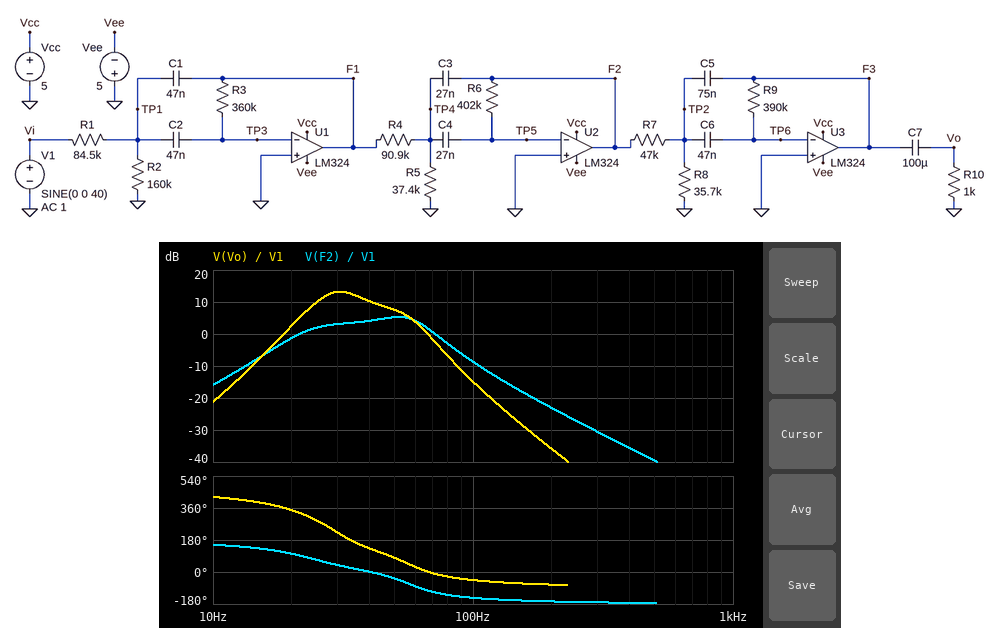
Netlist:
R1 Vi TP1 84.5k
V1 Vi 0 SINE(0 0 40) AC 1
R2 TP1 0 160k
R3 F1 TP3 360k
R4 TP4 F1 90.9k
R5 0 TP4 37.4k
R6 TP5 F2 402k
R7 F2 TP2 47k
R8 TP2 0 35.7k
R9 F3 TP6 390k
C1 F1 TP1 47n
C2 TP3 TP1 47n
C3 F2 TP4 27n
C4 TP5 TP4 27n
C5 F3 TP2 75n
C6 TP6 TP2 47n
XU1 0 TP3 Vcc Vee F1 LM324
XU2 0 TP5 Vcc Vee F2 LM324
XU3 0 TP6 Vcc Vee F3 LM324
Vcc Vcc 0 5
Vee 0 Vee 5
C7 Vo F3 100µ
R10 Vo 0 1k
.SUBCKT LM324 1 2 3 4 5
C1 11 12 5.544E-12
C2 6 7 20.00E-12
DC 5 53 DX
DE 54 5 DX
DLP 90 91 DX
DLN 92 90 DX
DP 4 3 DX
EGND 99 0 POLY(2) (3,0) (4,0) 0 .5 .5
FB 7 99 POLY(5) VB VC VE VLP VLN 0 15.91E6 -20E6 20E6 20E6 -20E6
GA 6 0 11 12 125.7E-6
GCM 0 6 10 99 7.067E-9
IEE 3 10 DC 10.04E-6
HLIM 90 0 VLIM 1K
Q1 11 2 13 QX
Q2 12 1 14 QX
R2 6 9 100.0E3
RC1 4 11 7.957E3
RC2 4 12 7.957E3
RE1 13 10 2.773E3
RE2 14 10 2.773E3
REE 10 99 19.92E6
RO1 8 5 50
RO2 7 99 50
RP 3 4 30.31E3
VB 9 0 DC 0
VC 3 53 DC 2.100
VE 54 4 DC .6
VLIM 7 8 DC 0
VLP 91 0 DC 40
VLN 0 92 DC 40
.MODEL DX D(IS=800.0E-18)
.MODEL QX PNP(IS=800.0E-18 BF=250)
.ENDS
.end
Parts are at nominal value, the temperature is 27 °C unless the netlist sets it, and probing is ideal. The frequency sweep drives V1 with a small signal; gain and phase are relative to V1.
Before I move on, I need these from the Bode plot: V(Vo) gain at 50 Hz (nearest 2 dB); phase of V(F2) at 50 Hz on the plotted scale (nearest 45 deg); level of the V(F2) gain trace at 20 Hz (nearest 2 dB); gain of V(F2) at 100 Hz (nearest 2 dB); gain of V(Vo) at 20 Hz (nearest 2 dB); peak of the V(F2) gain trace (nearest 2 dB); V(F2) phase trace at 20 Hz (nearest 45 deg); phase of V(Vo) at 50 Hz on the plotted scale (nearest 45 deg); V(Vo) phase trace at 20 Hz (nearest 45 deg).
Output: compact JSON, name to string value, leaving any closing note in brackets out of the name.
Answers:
{"V(Vo) gain at 50 Hz": "8 dB", "phase of V(F2) at 50 Hz on the plotted scale": "-45 deg", "level of the V(F2) gain trace at 20 Hz": "-2 dB", "gain of V(F2) at 100 Hz": "-8 dB", "gain of V(Vo) at 20 Hz": "2 dB", "peak of the V(F2) gain trace": "6 dB", "V(F2) phase trace at 20 Hz": "90 deg", "phase of V(Vo) at 50 Hz on the plotted scale": "90 deg", "V(Vo) phase trace at 20 Hz": "360 deg"}
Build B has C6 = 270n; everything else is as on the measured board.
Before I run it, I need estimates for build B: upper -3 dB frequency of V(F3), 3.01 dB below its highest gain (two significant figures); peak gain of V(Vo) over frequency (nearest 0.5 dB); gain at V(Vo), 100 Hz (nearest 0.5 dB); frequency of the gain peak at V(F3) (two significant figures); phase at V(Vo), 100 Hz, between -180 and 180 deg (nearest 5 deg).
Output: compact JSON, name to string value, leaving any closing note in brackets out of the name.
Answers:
{"upper -3 dB frequency of V(F3), 3.01 dB below its highest gain": "38 Hz", "peak gain of V(Vo) over frequency": "9.0 dB", "gain at V(Vo), 100 Hz": "-15.5 dB", "frequency of the gain peak at V(F3)": "23 Hz", "phase at V(Vo), 100 Hz, between -180 and 180 deg": "-50 deg"}
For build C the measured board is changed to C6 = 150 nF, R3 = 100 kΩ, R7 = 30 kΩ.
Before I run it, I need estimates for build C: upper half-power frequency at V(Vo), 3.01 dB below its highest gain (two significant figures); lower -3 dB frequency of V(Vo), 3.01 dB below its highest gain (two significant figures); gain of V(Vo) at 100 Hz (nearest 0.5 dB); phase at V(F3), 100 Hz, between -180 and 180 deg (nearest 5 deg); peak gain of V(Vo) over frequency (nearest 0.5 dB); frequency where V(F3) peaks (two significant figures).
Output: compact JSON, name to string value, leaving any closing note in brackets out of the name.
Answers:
{"upper half-power frequency at V(Vo), 3.01 dB below its highest gain": "64 Hz", "lower -3 dB frequency of V(Vo), 3.01 dB below its highest gain": "19 Hz", "gain of V(Vo) at 100 Hz": "-12.0 dB", "phase at V(F3), 100 Hz, between -180 and 180 deg": "-20 deg", "peak gain of V(Vo) over frequency": "5.5 dB", "frequency where V(F3) peaks": "51 Hz"}
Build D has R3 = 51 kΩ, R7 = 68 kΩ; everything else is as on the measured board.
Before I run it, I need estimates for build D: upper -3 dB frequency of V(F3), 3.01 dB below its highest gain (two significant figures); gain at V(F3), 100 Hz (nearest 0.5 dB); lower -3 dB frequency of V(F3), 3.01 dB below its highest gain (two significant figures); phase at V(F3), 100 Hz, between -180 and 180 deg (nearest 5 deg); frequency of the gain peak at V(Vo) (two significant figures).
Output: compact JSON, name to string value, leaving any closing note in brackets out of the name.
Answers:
{"upper -3 dB frequency of V(F3), 3.01 dB below its highest gain": "65 Hz", "gain at V(F3), 100 Hz": "-22.0 dB", "lower -3 dB frequency of V(F3), 3.01 dB below its highest gain": "28 Hz", "phase at V(F3), 100 Hz, between -180 and 180 deg": "10 deg", "frequency of the gain peak at V(Vo)": "51 Hz"}
